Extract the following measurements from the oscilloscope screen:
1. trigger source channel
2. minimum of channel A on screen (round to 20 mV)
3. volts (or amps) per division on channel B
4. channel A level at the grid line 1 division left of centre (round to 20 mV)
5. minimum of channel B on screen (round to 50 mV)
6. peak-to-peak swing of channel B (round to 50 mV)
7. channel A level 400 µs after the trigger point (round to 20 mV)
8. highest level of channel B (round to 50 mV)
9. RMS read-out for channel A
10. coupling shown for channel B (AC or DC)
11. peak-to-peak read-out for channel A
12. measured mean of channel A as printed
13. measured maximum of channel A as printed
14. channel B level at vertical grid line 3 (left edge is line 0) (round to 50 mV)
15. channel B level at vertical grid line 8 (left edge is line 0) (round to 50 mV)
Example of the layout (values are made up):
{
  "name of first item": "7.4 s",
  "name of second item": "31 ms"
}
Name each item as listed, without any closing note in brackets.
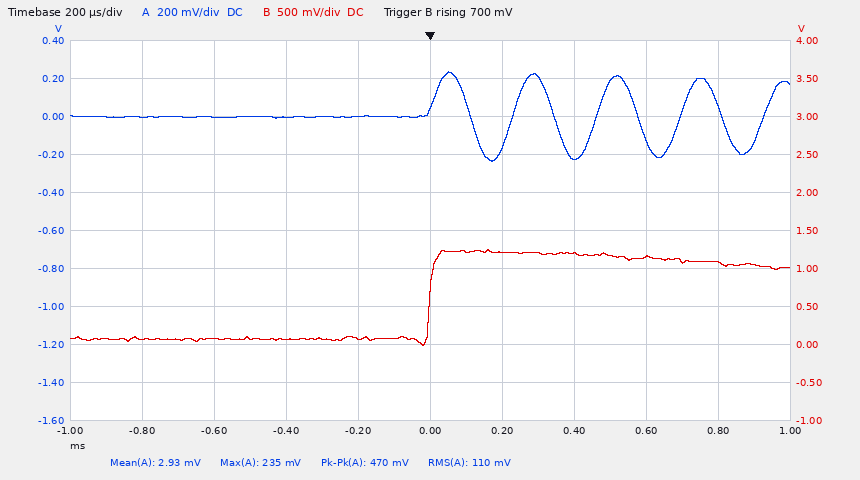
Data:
{
  "trigger source channel": "channel B",
  "minimum of channel A on screen": "-240 mV",
  "volts (or amps) per division on channel B": "500 mV",
  "channel A level at the grid line 1 division left of centre": "0 mV",
  "minimum of channel B on screen": "0 mV",
  "peak-to-peak swing of channel B": "1.25 V",
  "channel A level 400 µs after the trigger point": "-220 mV",
  "highest level of channel B": "1.25 V",
  "RMS read-out for channel A": "110 mV",
  "coupling shown for channel B": "DC",
  "peak-to-peak read-out for channel A": "470 mV",
  "measured mean of channel A as printed": "2.93 mV",
  "measured maximum of channel A as printed": "235 mV",
  "channel B level at vertical grid line 3 (left edge is line 0)": "50 mV",
  "channel B level at vertical grid line 8 (left edge is line 0)": "1.15 V"
}
